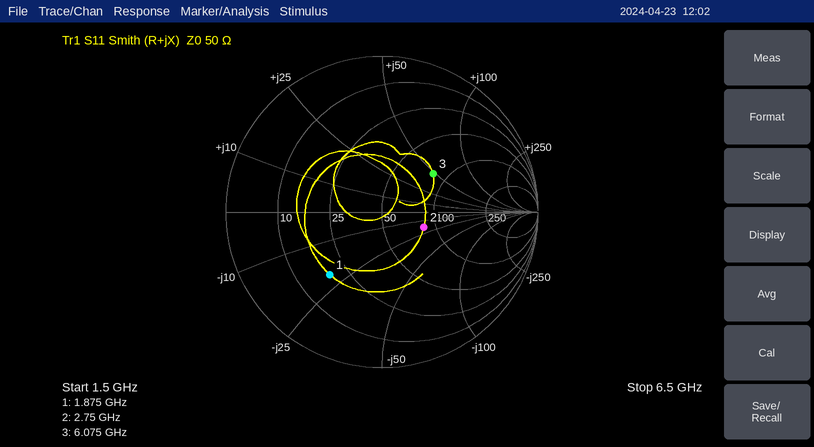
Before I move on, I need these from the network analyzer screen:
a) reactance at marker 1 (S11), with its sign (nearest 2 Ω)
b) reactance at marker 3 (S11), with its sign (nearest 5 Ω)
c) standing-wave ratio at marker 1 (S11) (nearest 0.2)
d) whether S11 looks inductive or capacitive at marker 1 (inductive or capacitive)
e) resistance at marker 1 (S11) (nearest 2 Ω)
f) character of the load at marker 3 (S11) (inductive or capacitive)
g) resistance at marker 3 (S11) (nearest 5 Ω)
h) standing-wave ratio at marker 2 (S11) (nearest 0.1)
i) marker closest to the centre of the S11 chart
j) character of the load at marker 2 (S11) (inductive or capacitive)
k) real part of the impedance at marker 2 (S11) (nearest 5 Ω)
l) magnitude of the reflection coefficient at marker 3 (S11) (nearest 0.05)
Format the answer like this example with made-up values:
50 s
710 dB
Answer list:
-20 Ω
+50 Ω
3.2
capacitive
18 Ω
inductive
80 Ω
1.8
marker 2
capacitive
85 Ω
0.40
